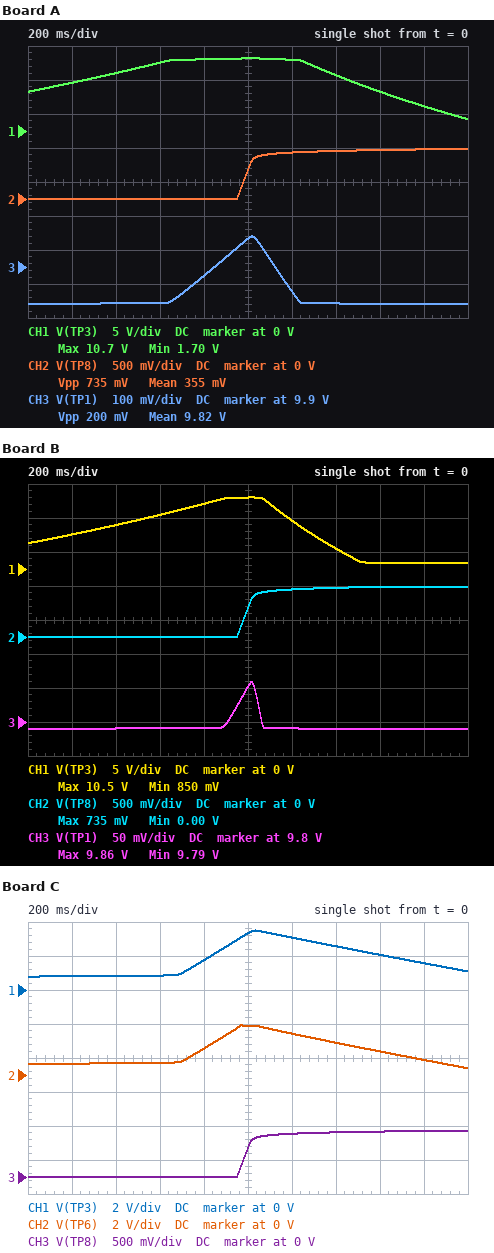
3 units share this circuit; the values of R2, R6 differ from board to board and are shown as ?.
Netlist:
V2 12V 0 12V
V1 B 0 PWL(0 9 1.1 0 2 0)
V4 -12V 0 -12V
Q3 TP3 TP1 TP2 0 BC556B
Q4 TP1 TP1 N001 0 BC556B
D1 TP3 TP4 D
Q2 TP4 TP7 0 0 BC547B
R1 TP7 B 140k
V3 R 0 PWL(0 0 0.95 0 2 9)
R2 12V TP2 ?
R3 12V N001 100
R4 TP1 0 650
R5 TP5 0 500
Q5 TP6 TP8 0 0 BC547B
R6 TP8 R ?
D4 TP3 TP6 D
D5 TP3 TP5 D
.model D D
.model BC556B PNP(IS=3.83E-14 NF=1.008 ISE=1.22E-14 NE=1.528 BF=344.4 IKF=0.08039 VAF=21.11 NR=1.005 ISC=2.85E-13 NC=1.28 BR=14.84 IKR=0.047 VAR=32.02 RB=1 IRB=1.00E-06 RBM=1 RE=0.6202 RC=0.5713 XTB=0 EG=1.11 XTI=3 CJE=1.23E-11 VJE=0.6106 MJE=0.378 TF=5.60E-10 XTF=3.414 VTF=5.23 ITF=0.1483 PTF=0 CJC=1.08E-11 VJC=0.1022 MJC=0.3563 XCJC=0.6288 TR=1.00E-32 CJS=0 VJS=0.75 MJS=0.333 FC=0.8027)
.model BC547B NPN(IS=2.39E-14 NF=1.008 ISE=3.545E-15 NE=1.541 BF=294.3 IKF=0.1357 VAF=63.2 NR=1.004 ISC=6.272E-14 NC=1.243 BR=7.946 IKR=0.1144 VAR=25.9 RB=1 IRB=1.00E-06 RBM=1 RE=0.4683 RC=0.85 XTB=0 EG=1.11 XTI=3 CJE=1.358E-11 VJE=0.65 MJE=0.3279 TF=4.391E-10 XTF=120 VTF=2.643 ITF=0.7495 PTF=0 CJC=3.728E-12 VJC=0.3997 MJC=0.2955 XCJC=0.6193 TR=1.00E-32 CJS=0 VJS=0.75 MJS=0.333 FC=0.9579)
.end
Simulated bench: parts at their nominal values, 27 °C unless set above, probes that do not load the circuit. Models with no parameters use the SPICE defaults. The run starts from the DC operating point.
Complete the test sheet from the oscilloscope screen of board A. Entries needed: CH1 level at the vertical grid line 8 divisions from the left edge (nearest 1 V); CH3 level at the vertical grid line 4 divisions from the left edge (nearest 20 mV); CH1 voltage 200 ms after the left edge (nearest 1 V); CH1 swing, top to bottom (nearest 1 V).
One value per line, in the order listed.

6 V
9.88 V
7 V
9 V
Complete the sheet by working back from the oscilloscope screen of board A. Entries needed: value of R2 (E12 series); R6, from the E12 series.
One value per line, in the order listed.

56 Ω
82 kΩ
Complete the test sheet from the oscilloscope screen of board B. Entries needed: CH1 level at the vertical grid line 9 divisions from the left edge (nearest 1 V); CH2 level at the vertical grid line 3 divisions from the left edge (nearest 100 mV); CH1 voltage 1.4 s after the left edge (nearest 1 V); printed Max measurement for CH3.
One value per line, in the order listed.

1 V
0 V
3 V
9.86 V
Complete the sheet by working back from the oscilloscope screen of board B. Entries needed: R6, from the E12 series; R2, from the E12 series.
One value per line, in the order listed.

47 kΩ
68 Ω
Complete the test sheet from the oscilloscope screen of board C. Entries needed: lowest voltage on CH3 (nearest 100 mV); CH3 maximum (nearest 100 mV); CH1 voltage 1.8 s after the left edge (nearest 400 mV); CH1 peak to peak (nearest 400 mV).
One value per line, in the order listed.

0 V
700 mV
1.6 V
2.8 V
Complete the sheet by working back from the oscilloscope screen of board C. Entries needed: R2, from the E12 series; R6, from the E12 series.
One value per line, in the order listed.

270 Ω
470 kΩ
